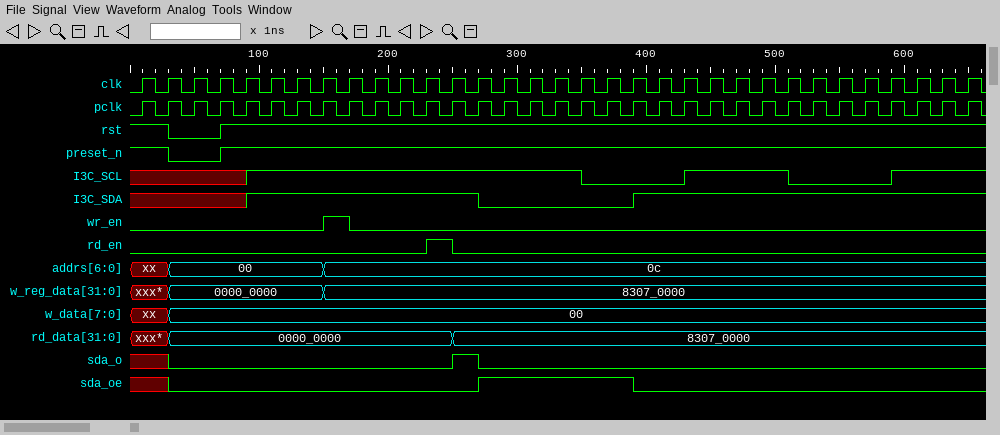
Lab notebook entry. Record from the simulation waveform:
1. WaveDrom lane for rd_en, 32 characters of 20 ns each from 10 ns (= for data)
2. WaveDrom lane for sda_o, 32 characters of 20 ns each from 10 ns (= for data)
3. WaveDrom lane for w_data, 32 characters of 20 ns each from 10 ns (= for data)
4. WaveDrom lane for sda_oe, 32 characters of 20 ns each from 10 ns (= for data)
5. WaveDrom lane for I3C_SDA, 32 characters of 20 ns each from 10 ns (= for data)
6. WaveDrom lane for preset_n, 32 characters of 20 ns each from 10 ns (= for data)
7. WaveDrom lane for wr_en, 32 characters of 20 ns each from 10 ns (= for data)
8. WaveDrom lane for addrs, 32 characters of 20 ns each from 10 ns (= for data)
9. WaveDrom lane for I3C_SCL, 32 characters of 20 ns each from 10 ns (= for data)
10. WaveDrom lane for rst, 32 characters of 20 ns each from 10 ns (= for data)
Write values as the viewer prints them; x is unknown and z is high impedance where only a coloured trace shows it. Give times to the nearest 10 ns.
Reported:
{name: 'rd_en', wave: '0..........10...................'}
{name: 'sda_o', wave: 'x0..........10..................'}
{name: 'w_data', wave: 'x=..............................', data: '00'}
{name: 'sda_oe', wave: 'x0...........1.....0............'}
{name: 'I3C_SDA', wave: 'x...1........0.....1............'}
{name: 'preset_n', wave: '10.1............................'}
{name: 'wr_en', wave: '0......10.......................'}
{name: 'addrs', wave: 'x=.....=........................', data: '00 0c'}
{name: 'I3C_SCL', wave: 'x...1............0...1...0...1..'}
{name: 'rst', wave: '10.1............................'}
